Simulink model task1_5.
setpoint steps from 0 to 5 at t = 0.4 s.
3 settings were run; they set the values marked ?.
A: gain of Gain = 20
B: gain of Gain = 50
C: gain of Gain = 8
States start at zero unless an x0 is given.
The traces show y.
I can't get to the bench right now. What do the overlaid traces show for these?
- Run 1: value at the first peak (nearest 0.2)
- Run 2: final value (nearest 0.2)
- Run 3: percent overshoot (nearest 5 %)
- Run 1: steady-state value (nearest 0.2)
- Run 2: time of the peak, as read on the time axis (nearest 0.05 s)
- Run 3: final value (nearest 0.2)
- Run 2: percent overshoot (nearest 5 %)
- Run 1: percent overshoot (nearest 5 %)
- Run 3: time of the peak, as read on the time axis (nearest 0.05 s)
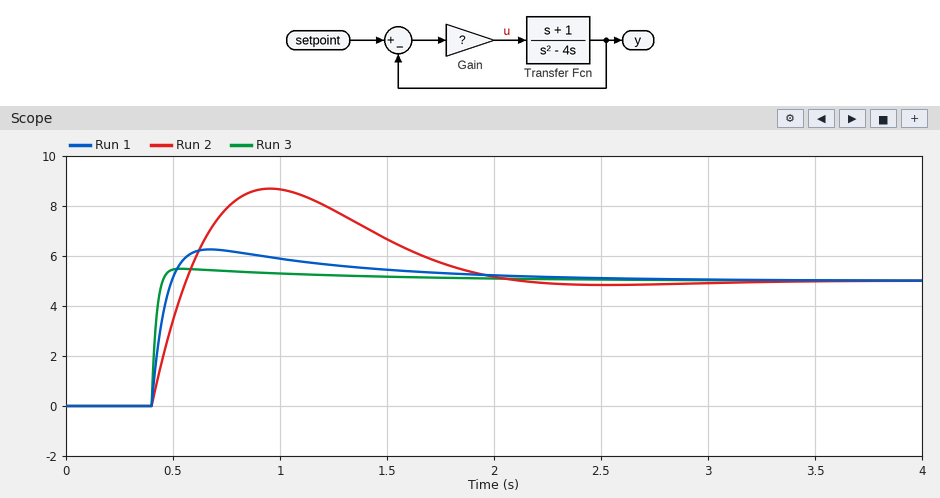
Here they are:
6.2
5.0
10 %
5.0
0.95 s
5.0
75 %
25 %
0.55 s
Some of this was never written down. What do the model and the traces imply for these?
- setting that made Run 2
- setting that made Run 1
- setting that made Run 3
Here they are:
C
A
B
